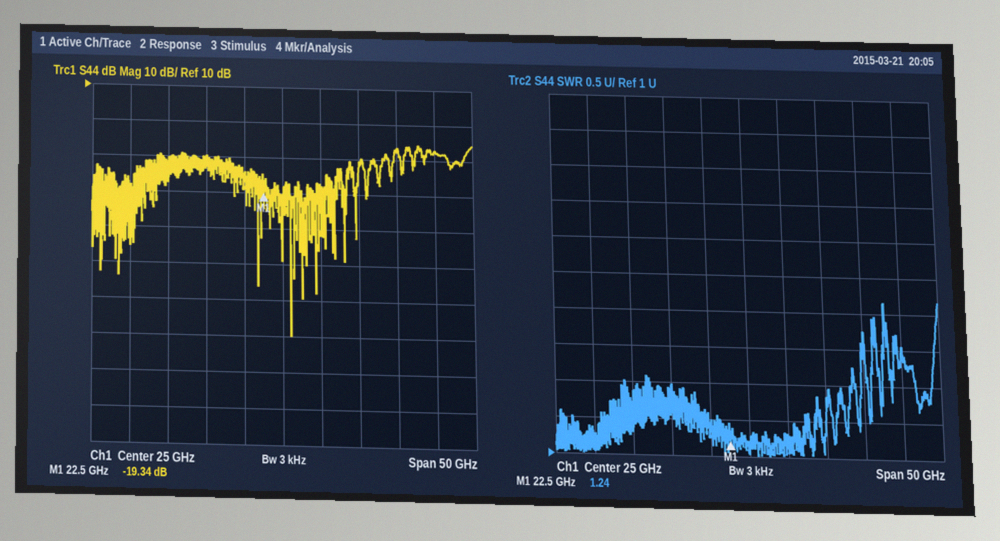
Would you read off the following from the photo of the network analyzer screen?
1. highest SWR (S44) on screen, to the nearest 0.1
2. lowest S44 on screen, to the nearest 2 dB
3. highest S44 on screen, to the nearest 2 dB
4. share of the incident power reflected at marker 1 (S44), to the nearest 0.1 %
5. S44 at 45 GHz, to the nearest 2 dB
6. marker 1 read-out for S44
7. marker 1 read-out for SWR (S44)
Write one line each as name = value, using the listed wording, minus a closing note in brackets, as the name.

highest SWR (S44) on screen, to the nearest 0.1 = 3.2
lowest S44 on screen, to the nearest 2 dB = -60 dB
highest S44 on screen, to the nearest 2 dB = -6 dB
share of the incident power reflected at marker 1 (S44), to the nearest 0.1 % = 1.2 %
S44 at 45 GHz, to the nearest 2 dB = -8 dB
marker 1 read-out for S44 = -19.34 dB
marker 1 read-out for SWR = 1.24
